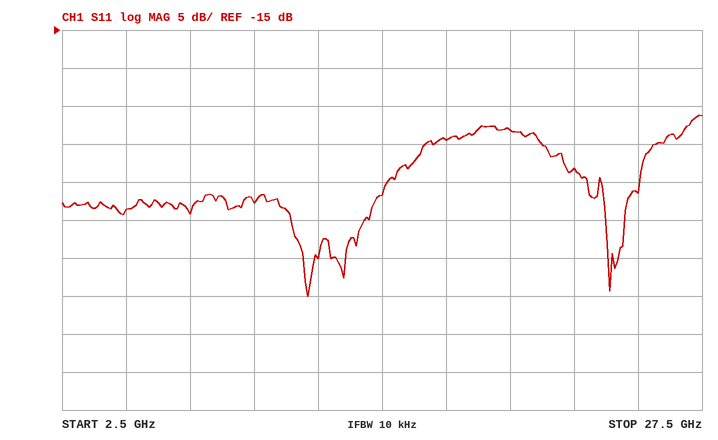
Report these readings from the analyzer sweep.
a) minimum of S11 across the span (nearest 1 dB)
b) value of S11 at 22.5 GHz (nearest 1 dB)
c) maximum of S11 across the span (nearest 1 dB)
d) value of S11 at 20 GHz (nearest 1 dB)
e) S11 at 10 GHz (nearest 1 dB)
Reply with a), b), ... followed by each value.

a) -50 dB
b) -33 dB
c) -26 dB
d) -28 dB
e) -38 dB
